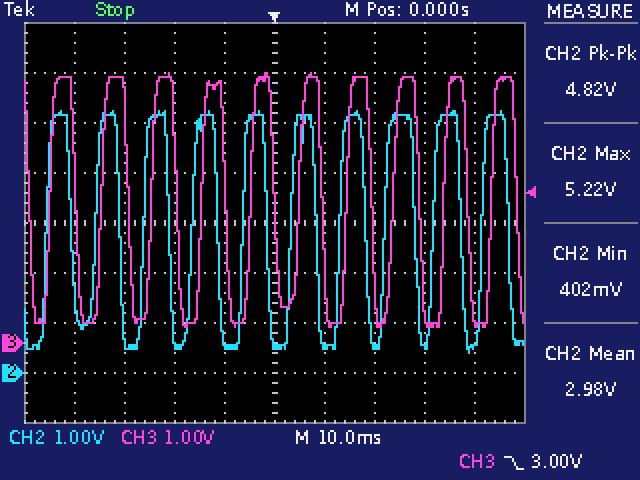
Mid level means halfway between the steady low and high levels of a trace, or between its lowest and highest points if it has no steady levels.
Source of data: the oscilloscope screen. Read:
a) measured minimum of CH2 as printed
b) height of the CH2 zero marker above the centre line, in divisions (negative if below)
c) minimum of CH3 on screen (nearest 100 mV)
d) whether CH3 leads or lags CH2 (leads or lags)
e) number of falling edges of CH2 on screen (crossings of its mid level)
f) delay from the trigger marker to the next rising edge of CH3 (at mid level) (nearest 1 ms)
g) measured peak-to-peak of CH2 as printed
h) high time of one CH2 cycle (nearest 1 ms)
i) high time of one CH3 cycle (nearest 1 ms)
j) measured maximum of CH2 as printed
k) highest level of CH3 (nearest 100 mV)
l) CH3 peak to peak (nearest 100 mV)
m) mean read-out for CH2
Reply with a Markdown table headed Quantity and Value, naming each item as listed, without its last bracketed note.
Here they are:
| Quantity | Value |
|---|---|
| measured minimum of CH2 as printed | 402 mV |
| height of the CH2 zero marker above the centre line, in divisions | -3.0 div |
| minimum of CH3 on screen | 300 mV |
| whether CH3 leads or lags CH2 | lags |
| number of falling edges of CH2 on screen | 10 |
| delay from the trigger marker to the next rising edge of CH3 (at mid level) | 5 ms |
| measured peak-to-peak of CH2 as printed | 4.82 V |
| high time of one CH2 cycle | 5 ms |
| high time of one CH3 cycle | 5 ms |
| measured maximum of CH2 as printed | 5.22 V |
| highest level of CH3 | 5.4 V |
| CH3 peak to peak | 5.1 V |
| mean read-out for CH2 | 2.98 V |
